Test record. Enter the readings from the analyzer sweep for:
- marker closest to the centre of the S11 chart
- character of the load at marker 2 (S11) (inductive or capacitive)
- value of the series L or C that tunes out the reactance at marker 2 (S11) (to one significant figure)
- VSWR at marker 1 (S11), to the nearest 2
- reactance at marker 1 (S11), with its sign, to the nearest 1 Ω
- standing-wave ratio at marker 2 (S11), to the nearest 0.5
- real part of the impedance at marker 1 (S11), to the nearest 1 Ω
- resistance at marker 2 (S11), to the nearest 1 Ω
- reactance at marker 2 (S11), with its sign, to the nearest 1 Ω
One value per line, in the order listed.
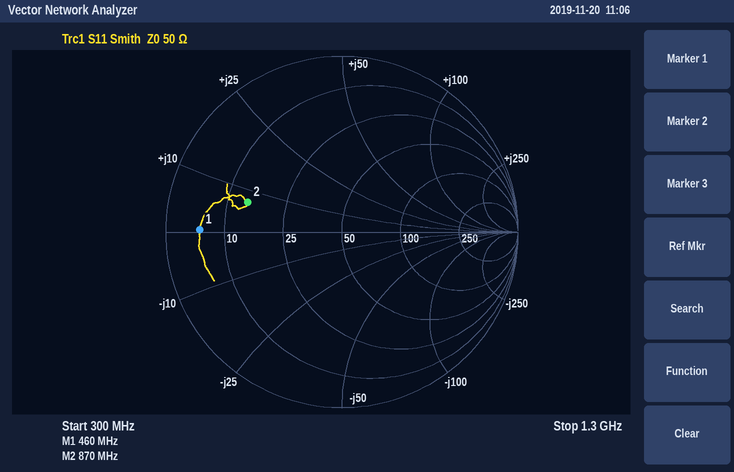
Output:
marker 2
inductive
30 pF
10
0 Ω
3.5
5 Ω
14 Ω
+7 Ω
